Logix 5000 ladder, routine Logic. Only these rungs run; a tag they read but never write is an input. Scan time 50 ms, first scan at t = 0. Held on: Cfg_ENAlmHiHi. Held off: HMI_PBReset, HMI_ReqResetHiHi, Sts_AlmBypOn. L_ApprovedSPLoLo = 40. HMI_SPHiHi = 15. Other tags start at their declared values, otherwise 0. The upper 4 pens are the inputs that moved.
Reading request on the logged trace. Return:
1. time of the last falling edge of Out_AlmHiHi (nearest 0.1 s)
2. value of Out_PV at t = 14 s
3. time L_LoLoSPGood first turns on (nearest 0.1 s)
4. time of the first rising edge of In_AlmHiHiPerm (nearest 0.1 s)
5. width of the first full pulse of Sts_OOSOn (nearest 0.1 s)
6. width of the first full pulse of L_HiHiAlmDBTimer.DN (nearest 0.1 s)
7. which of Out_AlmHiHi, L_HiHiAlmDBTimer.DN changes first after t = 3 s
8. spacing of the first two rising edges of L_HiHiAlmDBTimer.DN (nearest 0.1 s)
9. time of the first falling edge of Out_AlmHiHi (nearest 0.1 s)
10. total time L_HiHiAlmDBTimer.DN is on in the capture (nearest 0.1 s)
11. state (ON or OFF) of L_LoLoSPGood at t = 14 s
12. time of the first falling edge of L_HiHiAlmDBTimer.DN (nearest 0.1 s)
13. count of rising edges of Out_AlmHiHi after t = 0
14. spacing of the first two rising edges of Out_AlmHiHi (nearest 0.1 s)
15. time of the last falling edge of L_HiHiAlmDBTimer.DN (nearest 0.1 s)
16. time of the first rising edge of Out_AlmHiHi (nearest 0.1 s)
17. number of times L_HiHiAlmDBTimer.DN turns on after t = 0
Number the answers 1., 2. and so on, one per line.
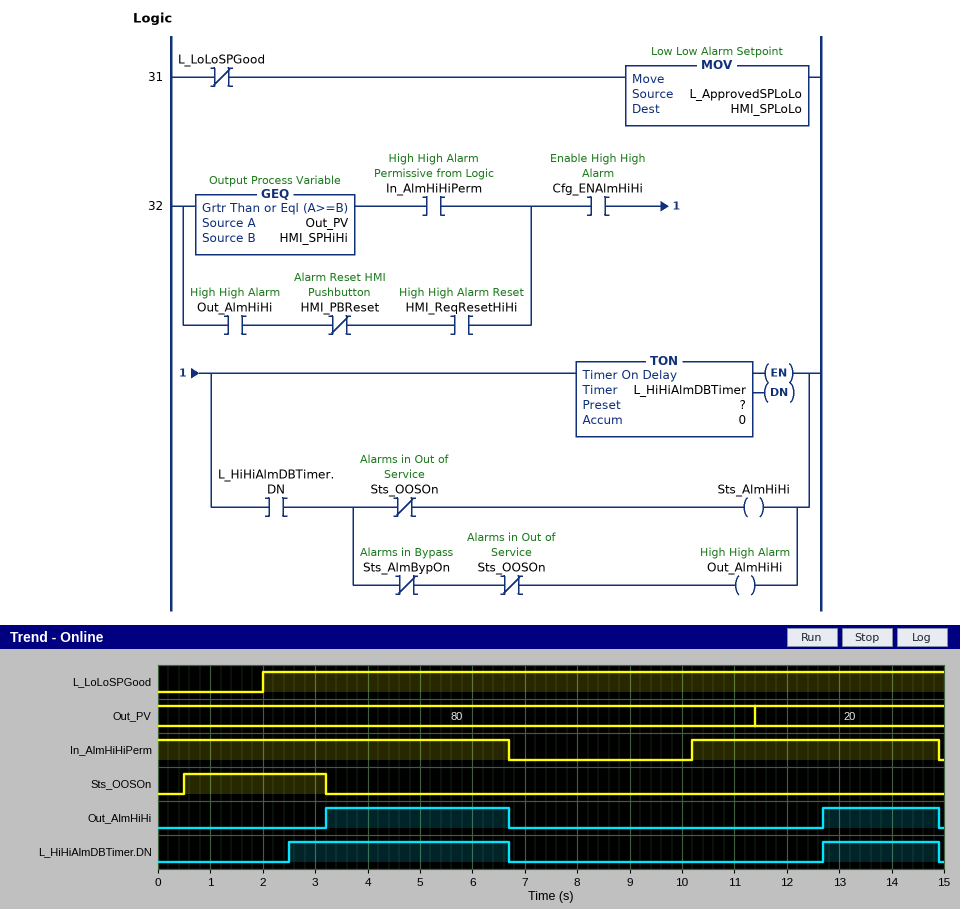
1. 14.9 s
2. 20
3. 2.0 s
4. 10.2 s
5. 2.7 s
6. 4.2 s
7. Out_AlmHiHi
8. 10.2 s
9. 6.7 s
10. 6.4 s
11. ON
12. 6.7 s
13. 2
14. 9.5 s
15. 14.9 s
16. 3.2 s
17. 2
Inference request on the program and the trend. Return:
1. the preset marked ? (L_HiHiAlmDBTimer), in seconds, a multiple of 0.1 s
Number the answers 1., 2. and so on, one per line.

1. 2.5 s
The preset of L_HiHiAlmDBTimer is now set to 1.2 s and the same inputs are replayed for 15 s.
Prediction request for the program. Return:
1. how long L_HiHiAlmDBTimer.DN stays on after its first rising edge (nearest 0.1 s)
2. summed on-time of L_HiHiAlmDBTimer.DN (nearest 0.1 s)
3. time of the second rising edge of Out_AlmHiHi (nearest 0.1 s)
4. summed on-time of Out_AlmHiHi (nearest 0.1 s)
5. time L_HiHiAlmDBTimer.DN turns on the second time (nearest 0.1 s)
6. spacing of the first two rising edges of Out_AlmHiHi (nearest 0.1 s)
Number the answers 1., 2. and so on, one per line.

1. 5.5 s
2. 9.0 s
3. 11.4 s
4. 7.0 s
5. 11.4 s
6. 8.2 s
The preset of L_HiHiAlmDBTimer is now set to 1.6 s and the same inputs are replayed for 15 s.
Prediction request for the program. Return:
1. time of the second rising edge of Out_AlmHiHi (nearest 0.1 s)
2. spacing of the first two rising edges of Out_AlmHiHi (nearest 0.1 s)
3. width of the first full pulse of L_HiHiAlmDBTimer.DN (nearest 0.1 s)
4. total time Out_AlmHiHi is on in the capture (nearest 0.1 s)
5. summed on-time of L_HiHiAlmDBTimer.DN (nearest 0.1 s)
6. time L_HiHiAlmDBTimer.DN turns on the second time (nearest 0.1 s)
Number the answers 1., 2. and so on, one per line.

1. 11.8 s
2. 8.6 s
3. 5.1 s
4. 6.6 s
5. 8.2 s
6. 11.8 s
